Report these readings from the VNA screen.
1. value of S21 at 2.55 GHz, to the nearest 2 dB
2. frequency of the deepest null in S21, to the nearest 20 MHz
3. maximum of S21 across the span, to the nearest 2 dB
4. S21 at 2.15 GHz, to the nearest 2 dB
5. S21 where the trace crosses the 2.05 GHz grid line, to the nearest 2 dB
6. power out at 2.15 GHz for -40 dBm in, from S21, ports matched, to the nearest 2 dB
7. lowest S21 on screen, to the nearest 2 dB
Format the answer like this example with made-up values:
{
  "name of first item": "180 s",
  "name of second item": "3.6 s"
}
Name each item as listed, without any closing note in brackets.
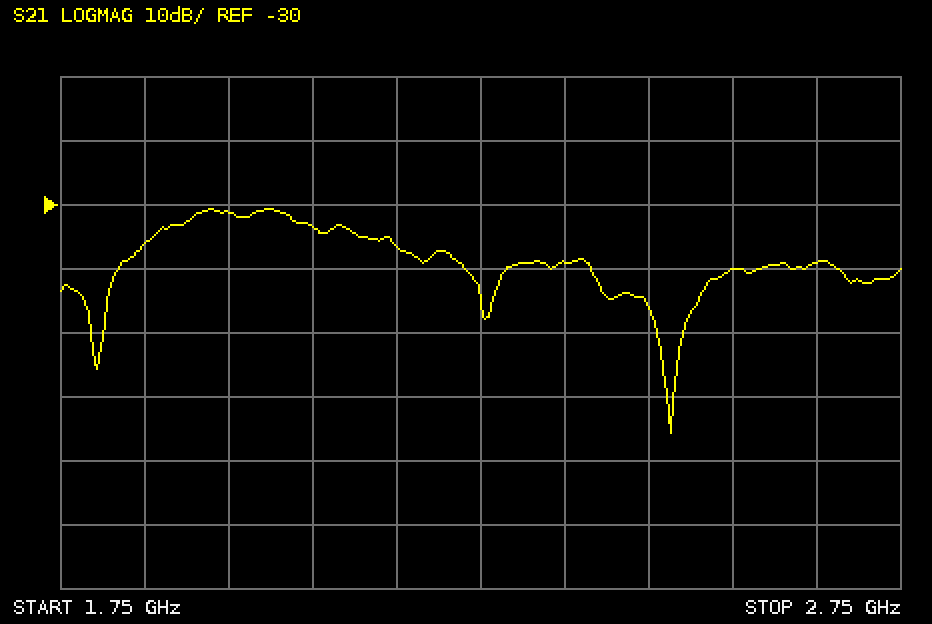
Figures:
{
  "value of S21 at 2.55 GHz, to the nearest 2 dB": "-40 dB",
  "frequency of the deepest null in S21, to the nearest 20 MHz": "2.48 GHz",
  "maximum of S21 across the span, to the nearest 2 dB": "-30 dB",
  "S21 at 2.15 GHz, to the nearest 2 dB": "-36 dB",
  "S21 where the trace crosses the 2.05 GHz grid line, to the nearest 2 dB": "-34 dB",
  "power out at 2.15 GHz for -40 dBm in, from S21, ports matched, to the nearest 2 dB": "-76 dBm",
  "lowest S21 on screen, to the nearest 2 dB": "-66 dB"
}
